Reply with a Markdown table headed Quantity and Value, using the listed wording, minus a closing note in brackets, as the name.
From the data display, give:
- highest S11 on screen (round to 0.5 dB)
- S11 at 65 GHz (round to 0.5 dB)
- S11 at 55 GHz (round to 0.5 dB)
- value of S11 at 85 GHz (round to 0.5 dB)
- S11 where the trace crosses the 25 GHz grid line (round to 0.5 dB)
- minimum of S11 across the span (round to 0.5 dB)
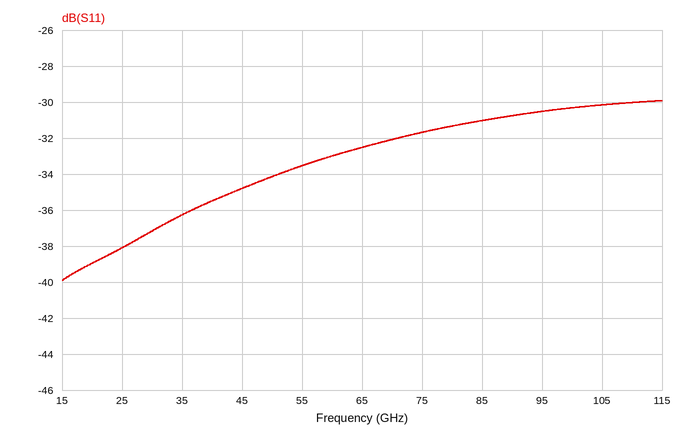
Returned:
| Quantity | Value |
|---|---|
| highest S11 on screen | -30.0 dB |
| S11 at 65 GHz | -32.5 dB |
| S11 at 55 GHz | -33.5 dB |
| value of S11 at 85 GHz | -31.0 dB |
| S11 where the trace crosses the 25 GHz grid line | -38.0 dB |
| minimum of S11 across the span | -40.0 dB |
